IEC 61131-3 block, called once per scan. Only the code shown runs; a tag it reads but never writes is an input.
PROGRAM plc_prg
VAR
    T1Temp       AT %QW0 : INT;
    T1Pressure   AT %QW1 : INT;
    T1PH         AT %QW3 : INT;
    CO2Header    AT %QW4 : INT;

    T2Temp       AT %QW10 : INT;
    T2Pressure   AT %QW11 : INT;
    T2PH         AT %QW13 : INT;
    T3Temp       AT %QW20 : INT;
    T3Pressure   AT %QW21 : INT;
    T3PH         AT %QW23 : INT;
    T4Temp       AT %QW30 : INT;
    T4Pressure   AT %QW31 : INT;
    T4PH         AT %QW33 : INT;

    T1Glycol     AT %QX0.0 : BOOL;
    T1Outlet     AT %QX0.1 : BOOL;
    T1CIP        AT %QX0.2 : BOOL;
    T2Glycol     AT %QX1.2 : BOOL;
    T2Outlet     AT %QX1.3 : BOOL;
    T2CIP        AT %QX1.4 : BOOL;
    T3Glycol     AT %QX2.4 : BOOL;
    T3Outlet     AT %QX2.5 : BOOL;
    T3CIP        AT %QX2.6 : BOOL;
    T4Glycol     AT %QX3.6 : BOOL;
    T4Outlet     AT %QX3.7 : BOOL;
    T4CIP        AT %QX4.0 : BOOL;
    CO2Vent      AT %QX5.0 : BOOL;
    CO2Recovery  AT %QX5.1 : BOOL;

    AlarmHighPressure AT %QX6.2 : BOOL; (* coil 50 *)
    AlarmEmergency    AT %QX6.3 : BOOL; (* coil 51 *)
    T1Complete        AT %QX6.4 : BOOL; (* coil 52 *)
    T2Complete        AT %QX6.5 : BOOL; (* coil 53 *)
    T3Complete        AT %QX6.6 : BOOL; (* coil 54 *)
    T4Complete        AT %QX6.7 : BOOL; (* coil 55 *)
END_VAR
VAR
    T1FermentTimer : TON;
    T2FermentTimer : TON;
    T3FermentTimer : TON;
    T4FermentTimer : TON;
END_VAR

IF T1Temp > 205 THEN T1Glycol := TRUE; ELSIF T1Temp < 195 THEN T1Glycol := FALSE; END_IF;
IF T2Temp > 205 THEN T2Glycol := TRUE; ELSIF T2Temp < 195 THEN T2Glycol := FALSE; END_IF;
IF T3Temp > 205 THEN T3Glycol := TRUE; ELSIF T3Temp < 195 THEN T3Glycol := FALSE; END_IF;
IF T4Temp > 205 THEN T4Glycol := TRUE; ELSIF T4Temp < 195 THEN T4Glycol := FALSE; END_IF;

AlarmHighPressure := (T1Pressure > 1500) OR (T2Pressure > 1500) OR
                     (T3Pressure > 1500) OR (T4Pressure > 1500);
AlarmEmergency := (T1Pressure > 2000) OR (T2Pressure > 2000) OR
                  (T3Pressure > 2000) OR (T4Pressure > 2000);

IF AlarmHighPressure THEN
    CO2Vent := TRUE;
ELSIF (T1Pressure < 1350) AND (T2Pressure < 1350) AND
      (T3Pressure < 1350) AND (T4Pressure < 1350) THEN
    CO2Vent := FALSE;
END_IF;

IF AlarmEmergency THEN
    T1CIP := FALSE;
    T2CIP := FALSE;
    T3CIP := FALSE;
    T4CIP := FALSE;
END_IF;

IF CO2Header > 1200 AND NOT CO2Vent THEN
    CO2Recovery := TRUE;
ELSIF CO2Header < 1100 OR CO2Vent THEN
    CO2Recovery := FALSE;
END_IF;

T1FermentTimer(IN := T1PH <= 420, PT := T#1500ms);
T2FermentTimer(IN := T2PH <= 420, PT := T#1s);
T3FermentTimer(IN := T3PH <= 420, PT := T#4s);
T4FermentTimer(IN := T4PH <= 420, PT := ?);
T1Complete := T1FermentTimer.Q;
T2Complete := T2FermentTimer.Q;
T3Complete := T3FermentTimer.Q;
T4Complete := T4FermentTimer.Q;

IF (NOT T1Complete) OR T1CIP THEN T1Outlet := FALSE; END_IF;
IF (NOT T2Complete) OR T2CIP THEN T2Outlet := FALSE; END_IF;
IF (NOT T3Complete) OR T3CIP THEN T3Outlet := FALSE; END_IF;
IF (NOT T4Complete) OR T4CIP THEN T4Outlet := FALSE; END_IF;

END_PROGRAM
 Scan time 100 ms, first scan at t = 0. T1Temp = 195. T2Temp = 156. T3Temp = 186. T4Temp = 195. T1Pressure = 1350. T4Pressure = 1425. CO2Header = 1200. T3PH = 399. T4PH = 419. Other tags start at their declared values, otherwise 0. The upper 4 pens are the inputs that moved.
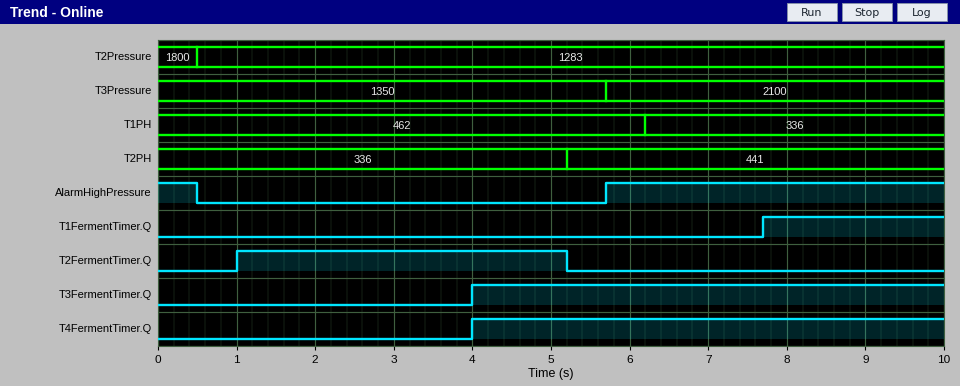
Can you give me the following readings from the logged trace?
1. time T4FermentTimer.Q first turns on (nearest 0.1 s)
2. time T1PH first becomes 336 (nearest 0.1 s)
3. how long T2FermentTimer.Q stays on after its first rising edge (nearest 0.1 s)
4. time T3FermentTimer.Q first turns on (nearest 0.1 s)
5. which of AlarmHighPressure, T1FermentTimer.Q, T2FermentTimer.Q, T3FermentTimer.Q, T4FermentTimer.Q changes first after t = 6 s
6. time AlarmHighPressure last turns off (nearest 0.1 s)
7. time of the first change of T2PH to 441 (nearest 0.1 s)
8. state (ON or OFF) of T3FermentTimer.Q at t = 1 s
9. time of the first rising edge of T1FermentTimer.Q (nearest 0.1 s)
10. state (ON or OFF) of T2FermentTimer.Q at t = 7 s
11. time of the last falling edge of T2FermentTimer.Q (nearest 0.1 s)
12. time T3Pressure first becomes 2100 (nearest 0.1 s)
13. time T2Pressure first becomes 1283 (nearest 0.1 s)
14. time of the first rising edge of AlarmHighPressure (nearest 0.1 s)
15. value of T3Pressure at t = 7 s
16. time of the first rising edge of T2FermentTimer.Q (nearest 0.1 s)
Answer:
4.0 s
6.2 s
4.2 s
4.0 s
T1FermentTimer.Q
0.5 s
5.2 s
OFF
7.7 s
OFF
5.2 s
5.7 s
0.5 s
5.7 s
2100
1.0 s
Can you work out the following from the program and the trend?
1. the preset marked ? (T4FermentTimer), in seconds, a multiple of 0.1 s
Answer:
4.0 s
